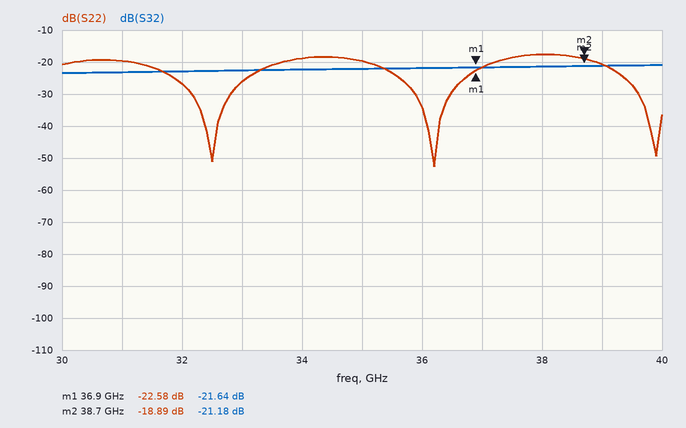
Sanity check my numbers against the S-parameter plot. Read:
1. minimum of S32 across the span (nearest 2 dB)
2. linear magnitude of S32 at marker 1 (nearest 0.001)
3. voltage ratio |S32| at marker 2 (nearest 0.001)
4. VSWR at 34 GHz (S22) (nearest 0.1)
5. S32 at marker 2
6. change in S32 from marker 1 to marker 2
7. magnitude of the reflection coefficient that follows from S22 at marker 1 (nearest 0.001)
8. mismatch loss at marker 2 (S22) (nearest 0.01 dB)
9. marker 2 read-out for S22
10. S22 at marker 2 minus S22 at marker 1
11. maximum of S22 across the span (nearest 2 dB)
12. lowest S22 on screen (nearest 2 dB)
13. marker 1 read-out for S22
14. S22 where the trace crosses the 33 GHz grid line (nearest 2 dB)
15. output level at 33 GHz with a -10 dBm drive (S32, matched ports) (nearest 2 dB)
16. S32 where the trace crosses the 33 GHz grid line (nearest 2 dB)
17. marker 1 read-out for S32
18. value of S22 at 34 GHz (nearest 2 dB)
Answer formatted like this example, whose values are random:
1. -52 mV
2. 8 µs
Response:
1. -24 dB
2. 0.083
3. 0.087
4. 1.3
5. -21.18 dB
6. 0.46 dB
7. 0.074
8. 0.06 dB
9. -18.89 dB
10. 3.69 dB
11. -18 dB
12. -52 dB
13. -22.58 dB
14. -26 dB
15. -32 dBm
16. -22 dB
17. -21.64 dB
18. -18 dB
